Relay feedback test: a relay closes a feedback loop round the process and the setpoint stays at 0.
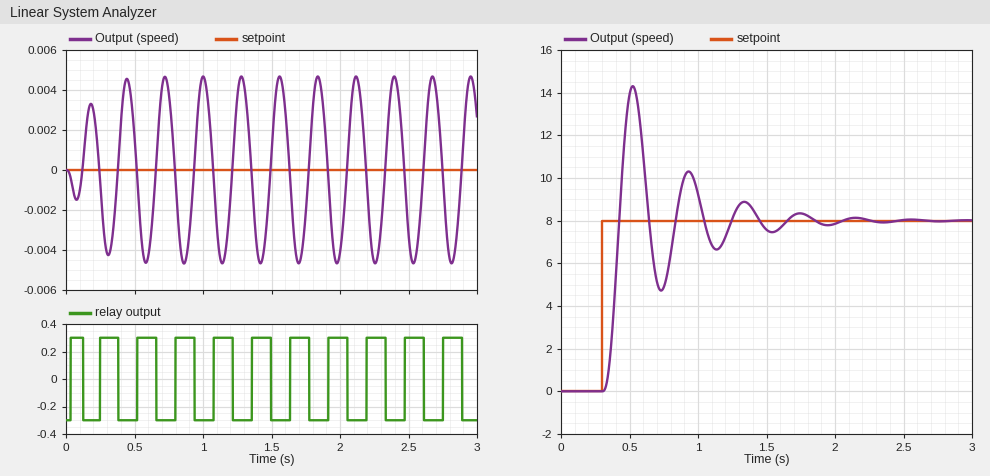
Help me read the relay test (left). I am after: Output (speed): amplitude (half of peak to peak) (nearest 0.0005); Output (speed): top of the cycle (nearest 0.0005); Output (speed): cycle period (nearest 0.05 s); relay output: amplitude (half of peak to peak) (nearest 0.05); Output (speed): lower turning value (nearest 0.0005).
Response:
0.0045
0.0045
0.30 s
0.30
-0.0045
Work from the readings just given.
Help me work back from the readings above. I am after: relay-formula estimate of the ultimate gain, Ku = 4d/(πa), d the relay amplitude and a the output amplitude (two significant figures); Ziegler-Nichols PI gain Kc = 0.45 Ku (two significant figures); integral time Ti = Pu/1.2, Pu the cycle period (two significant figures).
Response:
85
38
0.25 s
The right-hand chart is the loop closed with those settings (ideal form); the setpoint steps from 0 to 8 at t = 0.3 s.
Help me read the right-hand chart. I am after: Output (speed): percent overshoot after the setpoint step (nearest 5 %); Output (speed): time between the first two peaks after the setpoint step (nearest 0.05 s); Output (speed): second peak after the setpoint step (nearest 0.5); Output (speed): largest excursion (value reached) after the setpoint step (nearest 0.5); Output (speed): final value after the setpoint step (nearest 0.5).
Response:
80 %
0.40 s
10.5
14.5
8.0
